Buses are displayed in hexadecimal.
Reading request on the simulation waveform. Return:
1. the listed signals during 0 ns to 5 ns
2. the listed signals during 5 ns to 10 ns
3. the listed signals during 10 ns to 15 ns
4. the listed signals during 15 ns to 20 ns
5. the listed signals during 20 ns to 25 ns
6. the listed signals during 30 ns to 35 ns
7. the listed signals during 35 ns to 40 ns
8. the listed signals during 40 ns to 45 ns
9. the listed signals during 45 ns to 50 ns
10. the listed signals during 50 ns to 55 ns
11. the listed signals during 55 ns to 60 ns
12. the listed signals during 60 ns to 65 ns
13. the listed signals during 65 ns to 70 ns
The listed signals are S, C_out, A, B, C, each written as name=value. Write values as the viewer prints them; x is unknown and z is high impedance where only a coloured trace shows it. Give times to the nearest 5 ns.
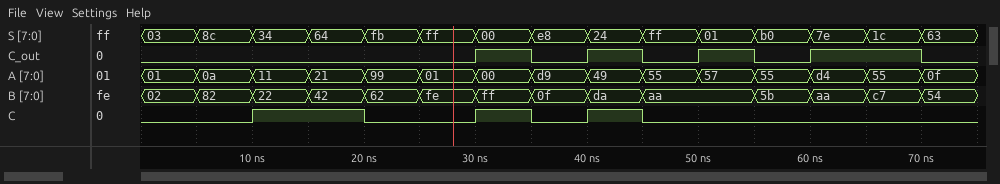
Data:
S=03, C_out=0, A=01, B=02, C=0
S=8c, C_out=0, A=0a, B=82, C=0
S=34, C_out=0, A=11, B=22, C=1
S=64, C_out=0, A=21, B=42, C=1
S=fb, C_out=0, A=99, B=62, C=0
S=00, C_out=1, A=00, B=ff, C=1
S=e8, C_out=0, A=d9, B=0f, C=0
S=24, C_out=1, A=49, B=da, C=1
S=ff, C_out=0, A=55, B=aa, C=0
S=01, C_out=1, A=57, B=aa, C=0
S=b0, C_out=0, A=55, B=5b, C=0
S=7e, C_out=1, A=d4, B=aa, C=0
S=1c, C_out=1, A=55, B=c7, C=0
